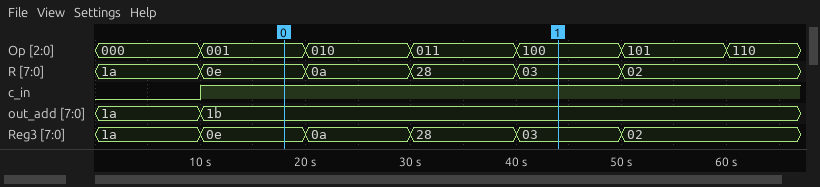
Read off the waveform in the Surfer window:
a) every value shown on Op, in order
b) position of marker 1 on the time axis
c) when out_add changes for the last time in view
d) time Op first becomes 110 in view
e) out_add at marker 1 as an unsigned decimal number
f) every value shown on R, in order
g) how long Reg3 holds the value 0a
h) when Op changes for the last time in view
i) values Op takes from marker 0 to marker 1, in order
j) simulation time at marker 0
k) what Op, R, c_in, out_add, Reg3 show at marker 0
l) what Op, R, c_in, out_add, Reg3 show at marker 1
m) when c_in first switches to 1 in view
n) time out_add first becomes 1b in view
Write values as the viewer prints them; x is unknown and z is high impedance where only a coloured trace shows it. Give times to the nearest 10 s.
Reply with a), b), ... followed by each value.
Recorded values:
a) 000, 001, 010, 011, 100, 101, 110
b) 40 s
c) 10 s
d) 60 s
e) 27
f) 1a, 0e, 0a, 28, 03, 02
g) 10 s
h) 60 s
i) 001, 010, 011, 100
j) 20 s
k) Op=001, R=0e, c_in=1, out_add=1b, Reg3=0e
l) Op=100, R=03, c_in=1, out_add=1b, Reg3=03
m) 10 s
n) 10 s
